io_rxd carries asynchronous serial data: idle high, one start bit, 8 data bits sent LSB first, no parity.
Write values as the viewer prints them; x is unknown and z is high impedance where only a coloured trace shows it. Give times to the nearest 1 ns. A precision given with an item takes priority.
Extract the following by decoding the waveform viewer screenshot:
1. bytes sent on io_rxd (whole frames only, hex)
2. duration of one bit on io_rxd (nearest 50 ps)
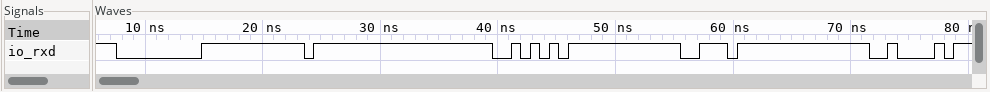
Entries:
00, FF, AA, EE, 42
800 ps
